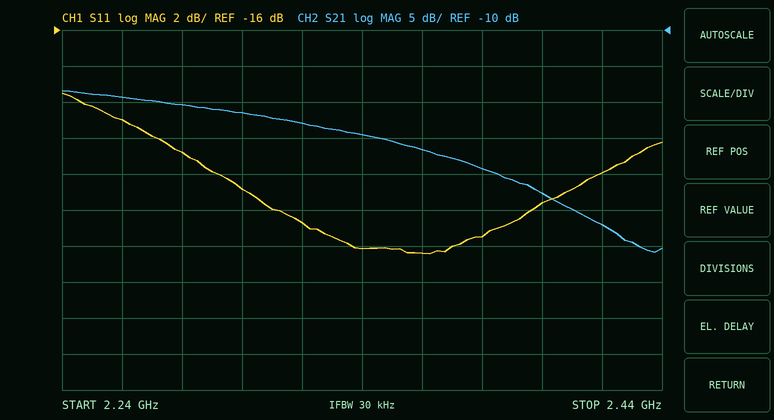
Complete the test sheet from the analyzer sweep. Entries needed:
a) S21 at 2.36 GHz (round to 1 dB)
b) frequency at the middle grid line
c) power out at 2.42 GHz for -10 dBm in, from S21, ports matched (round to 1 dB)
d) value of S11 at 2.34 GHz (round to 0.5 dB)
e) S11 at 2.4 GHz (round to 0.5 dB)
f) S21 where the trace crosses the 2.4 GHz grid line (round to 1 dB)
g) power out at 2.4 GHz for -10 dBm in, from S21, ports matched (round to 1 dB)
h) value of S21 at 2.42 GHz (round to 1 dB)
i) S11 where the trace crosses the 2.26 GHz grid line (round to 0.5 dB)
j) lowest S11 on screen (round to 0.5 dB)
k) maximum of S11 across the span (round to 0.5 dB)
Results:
-27 dB
2.34 GHz
-47 dBm
-28.0 dB
-25.5 dB
-33 dB
-43 dBm
-37 dB
-21.0 dB
-28.5 dB
-19.5 dB
